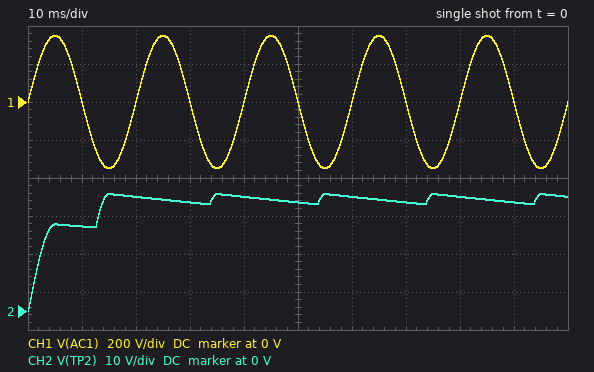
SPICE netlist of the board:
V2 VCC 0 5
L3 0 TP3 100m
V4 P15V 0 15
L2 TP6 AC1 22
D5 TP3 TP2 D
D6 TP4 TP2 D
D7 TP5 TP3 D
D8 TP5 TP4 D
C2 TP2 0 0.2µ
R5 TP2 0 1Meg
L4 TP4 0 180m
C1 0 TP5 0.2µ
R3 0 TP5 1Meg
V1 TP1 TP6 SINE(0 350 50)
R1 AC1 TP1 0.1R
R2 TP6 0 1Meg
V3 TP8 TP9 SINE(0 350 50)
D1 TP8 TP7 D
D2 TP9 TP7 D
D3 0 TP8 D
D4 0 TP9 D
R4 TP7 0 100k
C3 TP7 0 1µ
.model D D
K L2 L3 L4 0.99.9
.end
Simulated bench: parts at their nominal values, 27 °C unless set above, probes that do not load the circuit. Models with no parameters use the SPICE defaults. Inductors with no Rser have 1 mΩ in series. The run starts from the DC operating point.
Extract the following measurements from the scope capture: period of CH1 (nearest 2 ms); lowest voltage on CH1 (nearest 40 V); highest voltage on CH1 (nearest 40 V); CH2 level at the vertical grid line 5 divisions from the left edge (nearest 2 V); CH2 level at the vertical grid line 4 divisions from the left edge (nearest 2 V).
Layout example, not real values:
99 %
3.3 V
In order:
20 ms
-360 V
360 V
28 V
30 V
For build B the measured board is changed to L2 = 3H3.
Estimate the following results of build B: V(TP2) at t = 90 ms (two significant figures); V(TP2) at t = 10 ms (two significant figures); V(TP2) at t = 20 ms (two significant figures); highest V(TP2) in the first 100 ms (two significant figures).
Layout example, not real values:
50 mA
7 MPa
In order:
75 V
58 V
78 V
80 V
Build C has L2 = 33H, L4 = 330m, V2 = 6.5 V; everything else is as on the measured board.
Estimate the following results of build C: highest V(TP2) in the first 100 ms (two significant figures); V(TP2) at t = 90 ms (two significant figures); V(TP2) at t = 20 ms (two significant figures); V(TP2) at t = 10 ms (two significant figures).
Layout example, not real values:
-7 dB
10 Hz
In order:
34 V
32 V
33 V
18 V
